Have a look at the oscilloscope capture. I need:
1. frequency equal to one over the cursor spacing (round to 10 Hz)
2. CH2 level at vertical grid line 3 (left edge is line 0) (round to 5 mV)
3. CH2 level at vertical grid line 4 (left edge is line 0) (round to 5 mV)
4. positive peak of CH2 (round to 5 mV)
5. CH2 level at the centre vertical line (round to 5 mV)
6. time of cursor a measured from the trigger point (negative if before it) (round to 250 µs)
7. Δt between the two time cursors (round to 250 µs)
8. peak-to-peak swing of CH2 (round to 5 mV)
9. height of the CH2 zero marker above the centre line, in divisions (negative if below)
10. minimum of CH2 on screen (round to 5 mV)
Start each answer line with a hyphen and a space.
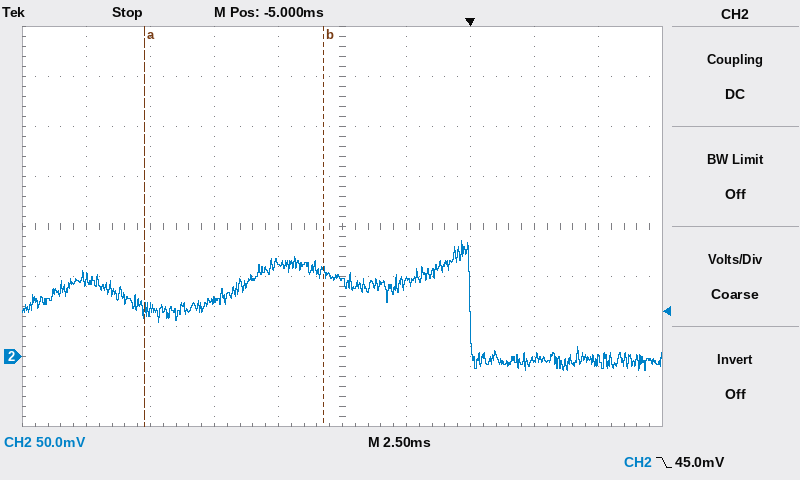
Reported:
- 140 Hz
- 55 mV
- 95 mV
- 115 mV
- 75 mV
- -12.75 ms
- 7.00 ms
- 130 mV
- -2.6 div
- -15 mV
